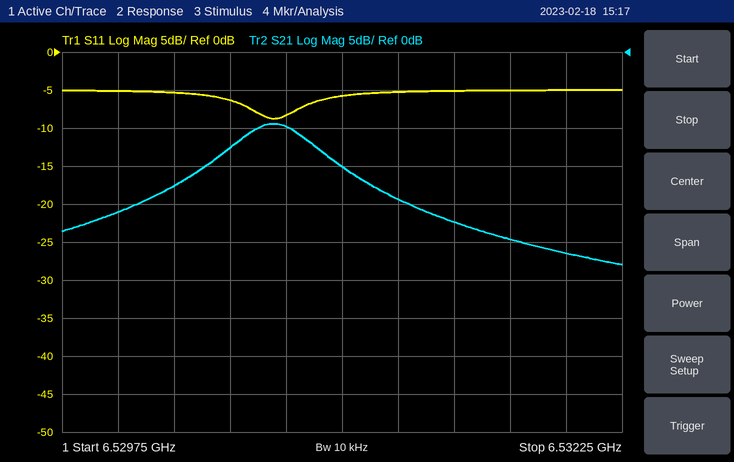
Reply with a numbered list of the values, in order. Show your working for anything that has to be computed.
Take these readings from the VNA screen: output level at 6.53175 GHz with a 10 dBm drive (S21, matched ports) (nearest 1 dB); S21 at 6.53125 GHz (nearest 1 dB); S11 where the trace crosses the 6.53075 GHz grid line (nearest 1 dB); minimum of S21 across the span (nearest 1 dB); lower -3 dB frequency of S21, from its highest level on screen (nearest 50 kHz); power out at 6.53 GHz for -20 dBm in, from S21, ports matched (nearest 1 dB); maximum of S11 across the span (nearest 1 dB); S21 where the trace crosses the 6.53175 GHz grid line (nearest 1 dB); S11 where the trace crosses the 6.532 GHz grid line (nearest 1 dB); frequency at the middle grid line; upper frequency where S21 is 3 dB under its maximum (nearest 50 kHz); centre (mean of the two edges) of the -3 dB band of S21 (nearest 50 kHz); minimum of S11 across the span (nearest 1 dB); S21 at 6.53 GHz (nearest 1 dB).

1. 10 dBm + (-25 dB) = -15 dBm
2. -19 dB
3. -8 dB
4. -28 dB
5. 6.53050 GHz
6. -20 dBm + (-21 dB) = -41 dBm
7. -5 dB
8. -25 dB
9. -5 dB
10. 6.531 GHz
11. 6.53090 GHz
12. 6.53070 GHz
13. -9 dB
14. -21 dB
